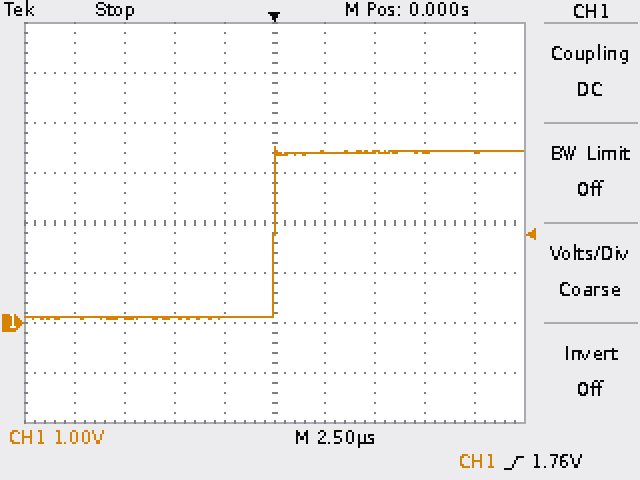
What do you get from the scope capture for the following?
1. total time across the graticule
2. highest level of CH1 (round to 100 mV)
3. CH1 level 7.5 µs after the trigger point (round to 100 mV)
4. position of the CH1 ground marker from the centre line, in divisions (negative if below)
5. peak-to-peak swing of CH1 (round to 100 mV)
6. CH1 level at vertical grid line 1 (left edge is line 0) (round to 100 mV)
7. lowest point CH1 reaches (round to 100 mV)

25 µs
3.5 V
3.4 V
-2.0 div
3.4 V
100 mV
100 mV
